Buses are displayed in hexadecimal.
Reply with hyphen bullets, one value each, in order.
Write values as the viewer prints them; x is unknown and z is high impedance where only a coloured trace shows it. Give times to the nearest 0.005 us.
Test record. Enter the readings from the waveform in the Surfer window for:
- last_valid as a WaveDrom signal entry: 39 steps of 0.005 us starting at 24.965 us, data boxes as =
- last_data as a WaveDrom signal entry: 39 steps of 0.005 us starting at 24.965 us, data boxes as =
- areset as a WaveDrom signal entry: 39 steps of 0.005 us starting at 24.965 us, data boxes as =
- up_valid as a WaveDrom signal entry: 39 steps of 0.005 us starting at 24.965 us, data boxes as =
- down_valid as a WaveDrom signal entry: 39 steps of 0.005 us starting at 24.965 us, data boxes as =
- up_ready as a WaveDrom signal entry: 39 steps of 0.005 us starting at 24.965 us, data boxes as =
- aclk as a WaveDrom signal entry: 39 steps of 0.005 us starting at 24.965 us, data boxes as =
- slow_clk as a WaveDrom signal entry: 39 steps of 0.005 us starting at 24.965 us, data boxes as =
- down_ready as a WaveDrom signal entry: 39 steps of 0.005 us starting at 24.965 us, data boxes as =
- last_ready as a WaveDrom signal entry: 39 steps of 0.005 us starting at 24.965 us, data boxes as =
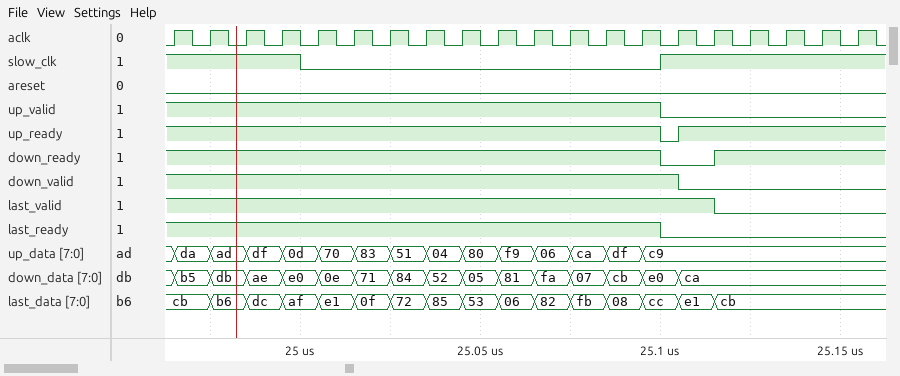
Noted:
- {name: 'last_valid', wave: '1.............................0........'}
- {name: 'last_data', wave: '=.=.=.=.=.=.=.=.=.=.=.=.=.=.=.=........', data: 'cb b6 dc af e1 0f 72 85 53 06 82 fb 08 cc e1 cb'}
- {name: 'areset', wave: '0......................................'}
- {name: 'up_valid', wave: '1..........................0...........'}
- {name: 'down_valid', wave: '1...........................0..........'}
- {name: 'up_ready', wave: '1..........................01..........'}
- {name: 'aclk', wave: '101010101010101010101010101010101010101'}
- {name: 'slow_clk', wave: '1......0...................1...........'}
- {name: 'down_ready', wave: '1..........................0..1........'}
- {name: 'last_ready', wave: '1..........................0...........'}
